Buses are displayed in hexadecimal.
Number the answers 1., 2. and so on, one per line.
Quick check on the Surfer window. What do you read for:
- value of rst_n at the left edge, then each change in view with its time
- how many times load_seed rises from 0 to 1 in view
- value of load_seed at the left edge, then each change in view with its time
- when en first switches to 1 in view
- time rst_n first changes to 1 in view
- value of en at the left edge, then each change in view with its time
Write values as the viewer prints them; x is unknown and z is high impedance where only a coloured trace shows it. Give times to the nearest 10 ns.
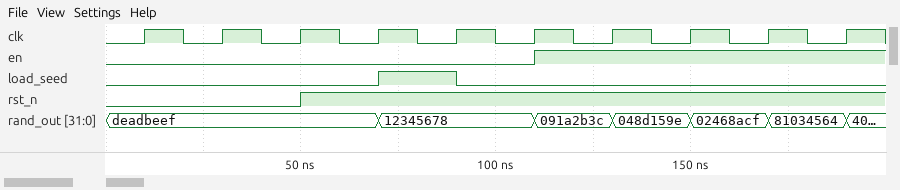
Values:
1. 0, 1 at 50 ns
2. 1
3. 0, 1 at 70 ns, 0 at 90 ns
4. 110 ns
5. 50 ns
6. 0, 1 at 110 ns
